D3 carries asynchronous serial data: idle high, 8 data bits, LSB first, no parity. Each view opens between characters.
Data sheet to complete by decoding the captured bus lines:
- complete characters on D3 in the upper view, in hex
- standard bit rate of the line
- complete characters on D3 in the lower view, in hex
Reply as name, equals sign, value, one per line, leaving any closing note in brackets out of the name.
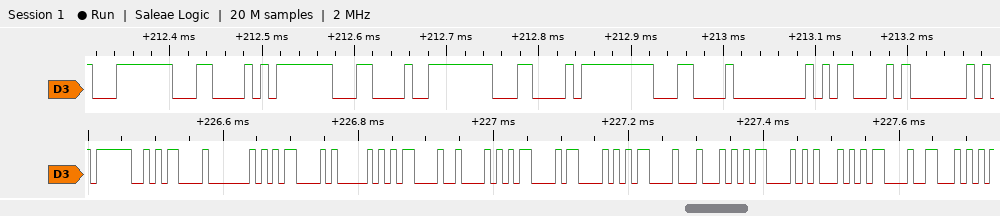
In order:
complete characters on D3 in the upper view, in hex = FC, 0C, FD, 0C, FE, 0C, FF, 0C, 00, 0D, 01
standard bit rate of the line = 115200 baud
complete characters on D3 in the lower view, in hex = 3F, 0D, 40, 0D, 41, 0D, 42, 0D, 43, 0D, 44, 0D, 45, 0D, 46
